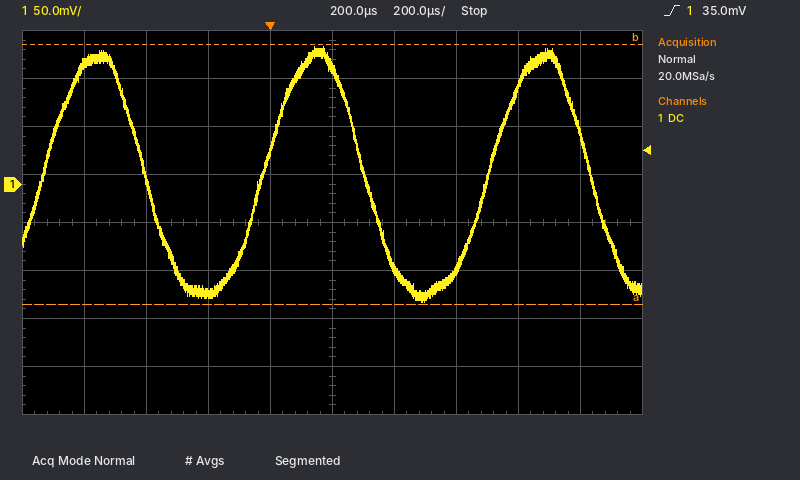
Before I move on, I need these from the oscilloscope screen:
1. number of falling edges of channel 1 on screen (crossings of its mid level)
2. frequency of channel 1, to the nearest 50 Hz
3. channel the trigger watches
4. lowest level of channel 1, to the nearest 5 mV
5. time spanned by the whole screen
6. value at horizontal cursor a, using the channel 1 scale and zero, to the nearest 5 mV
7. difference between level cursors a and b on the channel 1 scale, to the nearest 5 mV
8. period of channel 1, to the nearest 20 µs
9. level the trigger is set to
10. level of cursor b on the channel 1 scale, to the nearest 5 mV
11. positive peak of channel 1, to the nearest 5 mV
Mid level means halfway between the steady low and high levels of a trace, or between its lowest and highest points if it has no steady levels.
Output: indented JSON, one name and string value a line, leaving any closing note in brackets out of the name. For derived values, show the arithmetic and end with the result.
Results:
{
  "number of falling edges of channel 1 on screen": "3",
  "frequency of channel 1, to the nearest 50 Hz": "1 / 720 µs ≈ 1.39 kHz, so 1.40 kHz to the nearest 50 Hz",
  "channel the trigger watches": "channel 1",
  "lowest level of channel 1, to the nearest 5 mV": "-125 mV",
  "time spanned by the whole screen": "2 ms",
  "value at horizontal cursor a, using the channel 1 scale and zero, to the nearest 5 mV": "-125 mV",
  "difference between level cursors a and b on the channel 1 scale, to the nearest 5 mV": "270 mV",
  "period of channel 1, to the nearest 20 µs": "720 µs",
  "level the trigger is set to": "35.0 mV",
  "level of cursor b on the channel 1 scale, to the nearest 5 mV": "145 mV",
  "positive peak of channel 1, to the nearest 5 mV": "145 mV"
}
